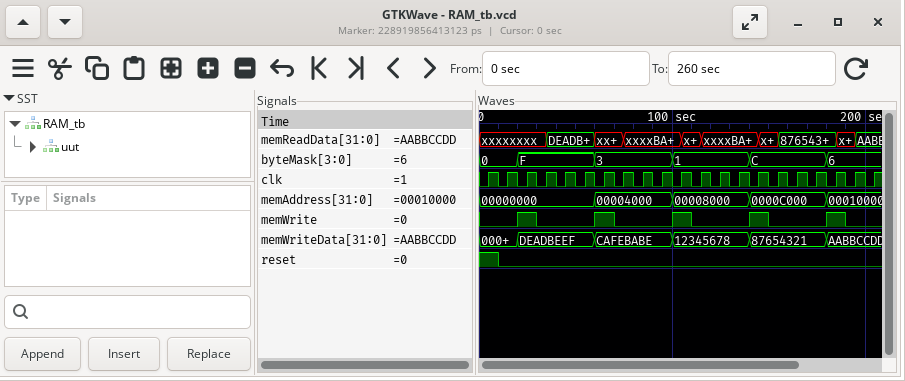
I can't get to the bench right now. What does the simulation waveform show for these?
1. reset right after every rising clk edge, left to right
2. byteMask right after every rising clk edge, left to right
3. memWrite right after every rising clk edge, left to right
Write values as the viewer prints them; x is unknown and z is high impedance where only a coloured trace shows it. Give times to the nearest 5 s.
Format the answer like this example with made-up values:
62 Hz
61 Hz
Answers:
1 0 0 0 0 0 0 0 0 0 0 0 0 0 0 0 0 0 0 0 0
0, 0, F, F, F, F, 3, 3, 3, 3, 1, 1, 1, 1, C, C, C, C, 6, 6, 6
0 0 1 0 0 0 1 0 0 0 1 0 0 0 1 0 0 0 1 0 0
